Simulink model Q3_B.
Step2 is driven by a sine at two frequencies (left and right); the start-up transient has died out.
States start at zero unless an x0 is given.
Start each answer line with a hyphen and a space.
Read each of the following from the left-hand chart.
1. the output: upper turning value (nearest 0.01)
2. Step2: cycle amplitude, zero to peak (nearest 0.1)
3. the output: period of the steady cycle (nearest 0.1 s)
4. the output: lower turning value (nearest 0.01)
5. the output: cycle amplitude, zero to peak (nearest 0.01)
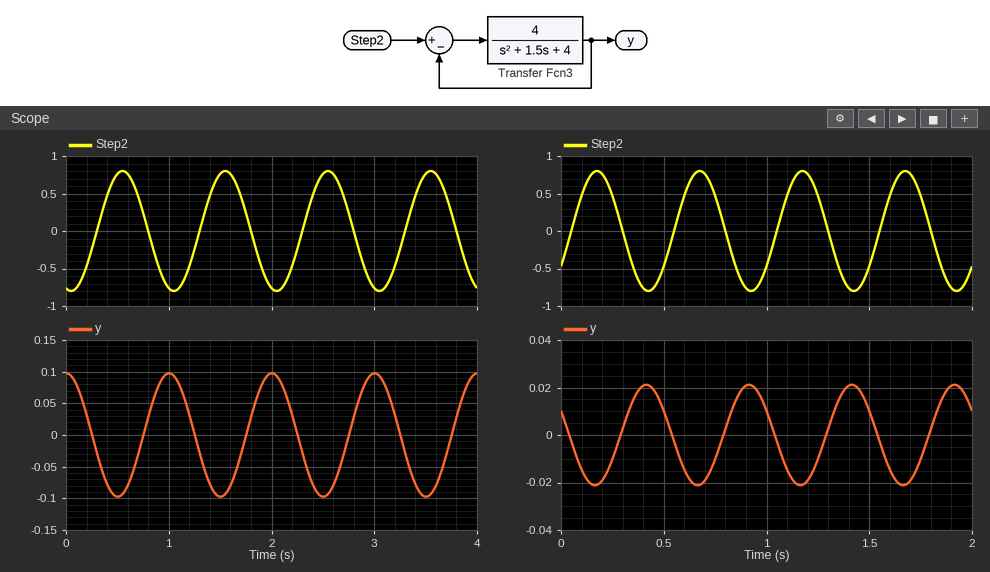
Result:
- 0.10
- 0.8
- 1.0 s
- -0.10
- 0.10
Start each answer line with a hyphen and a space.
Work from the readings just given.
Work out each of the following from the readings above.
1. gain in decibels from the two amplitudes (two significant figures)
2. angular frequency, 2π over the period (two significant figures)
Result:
- -18 dB
- 6.3 rad/s
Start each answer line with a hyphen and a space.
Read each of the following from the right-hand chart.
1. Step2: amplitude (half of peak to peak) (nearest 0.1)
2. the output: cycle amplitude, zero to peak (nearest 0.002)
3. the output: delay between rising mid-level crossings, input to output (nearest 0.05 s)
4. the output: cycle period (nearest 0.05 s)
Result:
- 0.8
- 0.022
- 0.25 s
- 0.50 s
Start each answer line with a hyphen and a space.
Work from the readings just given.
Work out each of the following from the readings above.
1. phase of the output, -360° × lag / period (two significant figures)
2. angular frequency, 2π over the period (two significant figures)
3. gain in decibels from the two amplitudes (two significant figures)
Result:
- -180°
- 13 rad/s
- -31 dB
